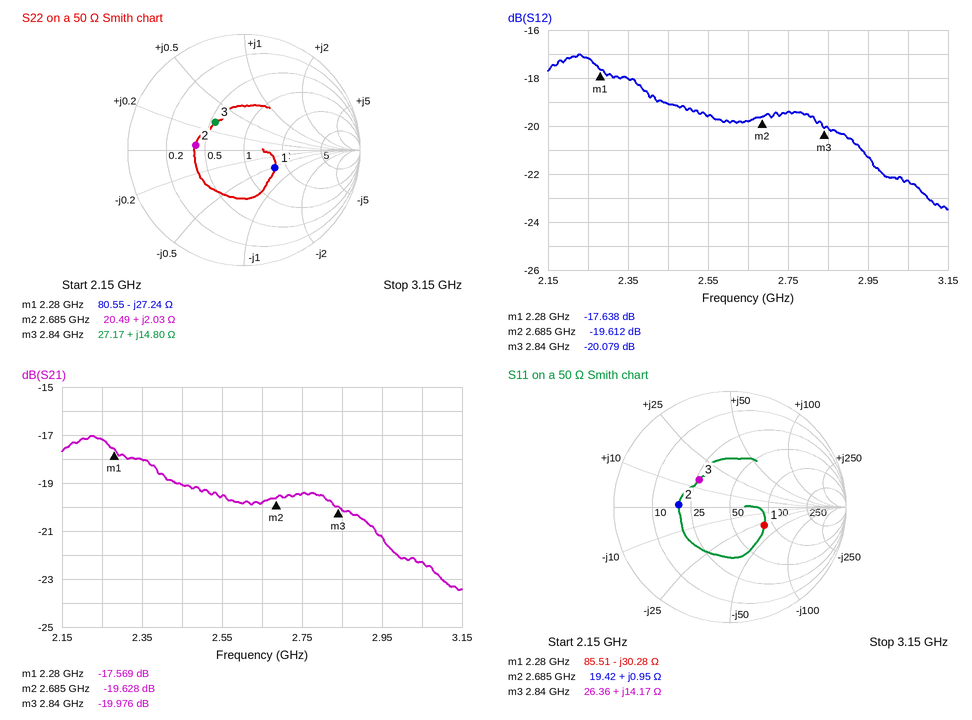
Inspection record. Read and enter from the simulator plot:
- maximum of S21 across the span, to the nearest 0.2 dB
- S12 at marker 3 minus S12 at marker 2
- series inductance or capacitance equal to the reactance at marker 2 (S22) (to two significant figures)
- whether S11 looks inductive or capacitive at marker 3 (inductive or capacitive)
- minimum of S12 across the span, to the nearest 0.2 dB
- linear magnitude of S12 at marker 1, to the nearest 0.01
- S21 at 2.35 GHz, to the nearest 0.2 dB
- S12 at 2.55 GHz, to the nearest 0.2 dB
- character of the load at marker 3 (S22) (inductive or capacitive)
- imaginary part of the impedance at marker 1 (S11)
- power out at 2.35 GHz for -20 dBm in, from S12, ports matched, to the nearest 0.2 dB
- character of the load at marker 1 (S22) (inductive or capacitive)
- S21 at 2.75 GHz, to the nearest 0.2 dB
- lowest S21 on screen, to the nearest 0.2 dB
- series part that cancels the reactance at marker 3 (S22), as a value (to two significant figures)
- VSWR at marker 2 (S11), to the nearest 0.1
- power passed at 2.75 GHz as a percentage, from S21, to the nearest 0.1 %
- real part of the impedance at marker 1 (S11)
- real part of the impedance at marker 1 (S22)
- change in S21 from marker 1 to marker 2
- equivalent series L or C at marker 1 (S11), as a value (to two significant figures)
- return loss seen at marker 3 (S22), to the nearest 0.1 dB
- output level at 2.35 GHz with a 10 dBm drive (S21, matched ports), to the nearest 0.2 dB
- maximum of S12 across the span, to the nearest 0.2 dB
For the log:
-17.0 dB
-0.467 dB
120 pH
inductive
-23.4 dB
0.13
-18.0 dB
-19.6 dB
inductive
-30.28 Ω
-38.0 dBm
capacitive
-19.4 dB
-23.4 dB
3.8 pF
2.6
1.1 %
85.51 Ω
80.55 Ω
-2.059 dB
2.3 pF
9.2 dB
-8.0 dBm
-17.0 dB
